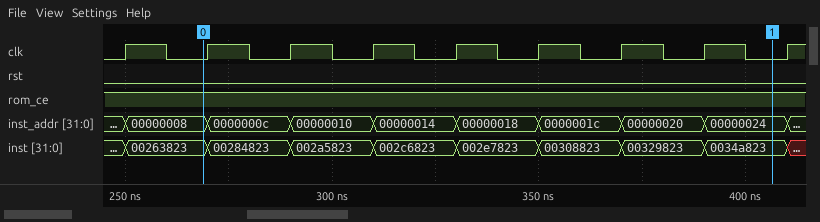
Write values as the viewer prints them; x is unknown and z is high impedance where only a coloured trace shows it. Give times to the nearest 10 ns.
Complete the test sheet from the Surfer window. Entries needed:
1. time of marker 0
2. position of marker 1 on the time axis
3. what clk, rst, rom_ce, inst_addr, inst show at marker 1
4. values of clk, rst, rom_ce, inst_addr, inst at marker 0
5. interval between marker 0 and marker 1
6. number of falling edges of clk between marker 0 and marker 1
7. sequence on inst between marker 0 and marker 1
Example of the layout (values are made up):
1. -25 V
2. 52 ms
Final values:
1. 270 ns
2. 410 ns
3. clk=0, rst=0, rom_ce=1, inst_addr=00000024, inst=0034a823
4. clk=0, rst=0, rom_ce=1, inst_addr=00000008, inst=00263823
5. 140 ns
6. 7
7. 00263823, 00284823, 002a5823, 002c6823, 002e7823, 00308823, 00329823, 0034a823
